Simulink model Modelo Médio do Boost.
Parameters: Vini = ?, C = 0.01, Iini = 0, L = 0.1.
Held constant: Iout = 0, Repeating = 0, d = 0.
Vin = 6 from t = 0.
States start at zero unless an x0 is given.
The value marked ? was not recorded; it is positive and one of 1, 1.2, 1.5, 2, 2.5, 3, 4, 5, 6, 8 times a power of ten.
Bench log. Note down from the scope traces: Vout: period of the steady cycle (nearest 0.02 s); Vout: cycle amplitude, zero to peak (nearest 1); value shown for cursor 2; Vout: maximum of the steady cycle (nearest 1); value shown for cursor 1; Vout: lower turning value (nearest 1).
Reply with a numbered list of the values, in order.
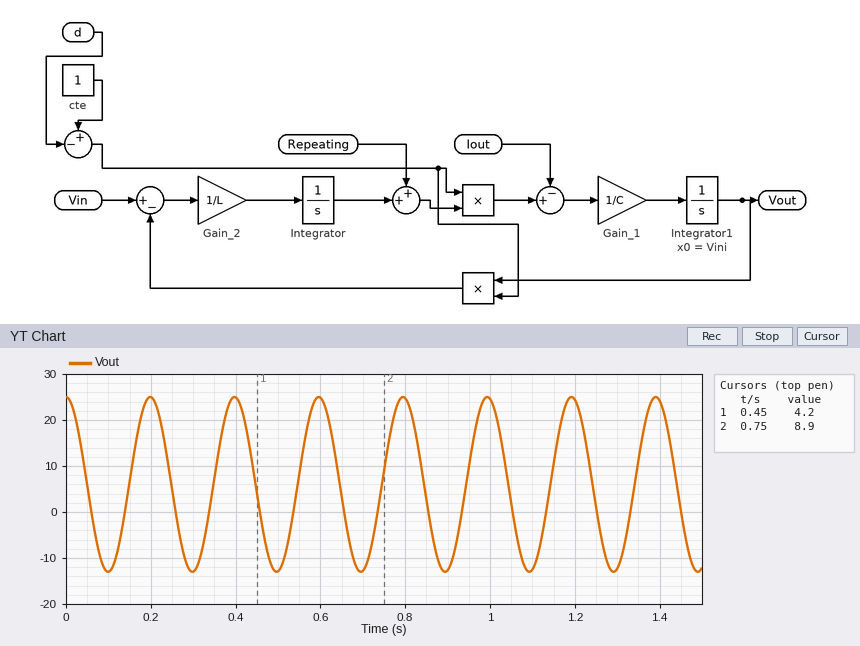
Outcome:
1. 0.20 s
2. 19
3. 8.9
4. 25
5. 4.2
6. -13
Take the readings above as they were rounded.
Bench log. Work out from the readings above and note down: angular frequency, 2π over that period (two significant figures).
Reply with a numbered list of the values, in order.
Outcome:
1. 31 rad/s
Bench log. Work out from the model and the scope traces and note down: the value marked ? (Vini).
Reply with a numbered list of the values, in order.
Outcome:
1. 25
